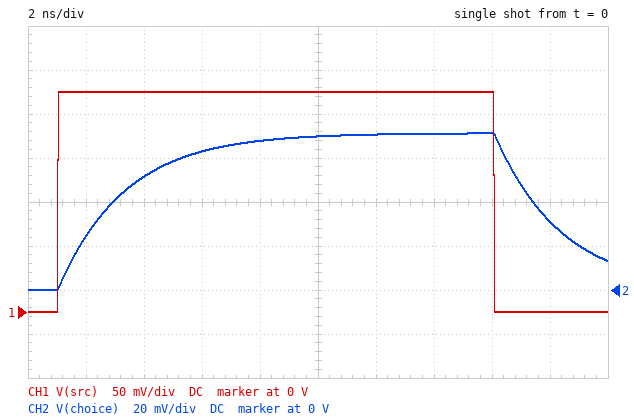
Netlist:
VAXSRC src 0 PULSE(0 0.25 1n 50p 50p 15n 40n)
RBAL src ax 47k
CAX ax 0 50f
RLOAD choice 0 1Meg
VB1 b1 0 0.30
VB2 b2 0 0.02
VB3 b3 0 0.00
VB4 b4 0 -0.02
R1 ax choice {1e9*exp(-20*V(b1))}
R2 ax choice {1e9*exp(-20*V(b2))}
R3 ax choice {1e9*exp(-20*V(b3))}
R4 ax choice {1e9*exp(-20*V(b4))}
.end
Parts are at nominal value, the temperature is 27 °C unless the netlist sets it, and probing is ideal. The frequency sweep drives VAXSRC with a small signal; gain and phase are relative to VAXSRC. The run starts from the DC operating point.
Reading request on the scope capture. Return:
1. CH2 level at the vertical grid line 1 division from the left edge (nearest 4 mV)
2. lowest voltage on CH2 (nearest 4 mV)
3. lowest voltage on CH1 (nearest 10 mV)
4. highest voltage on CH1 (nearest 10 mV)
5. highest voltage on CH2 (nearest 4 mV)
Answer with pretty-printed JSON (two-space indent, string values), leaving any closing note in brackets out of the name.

{
  "CH2 level at the vertical grid line 1 division from the left edge": "24 mV",
  "lowest voltage on CH2": "0 V",
  "lowest voltage on CH1": "0 V",
  "highest voltage on CH1": "250 mV",
  "highest voltage on CH2": "72 mV"
}
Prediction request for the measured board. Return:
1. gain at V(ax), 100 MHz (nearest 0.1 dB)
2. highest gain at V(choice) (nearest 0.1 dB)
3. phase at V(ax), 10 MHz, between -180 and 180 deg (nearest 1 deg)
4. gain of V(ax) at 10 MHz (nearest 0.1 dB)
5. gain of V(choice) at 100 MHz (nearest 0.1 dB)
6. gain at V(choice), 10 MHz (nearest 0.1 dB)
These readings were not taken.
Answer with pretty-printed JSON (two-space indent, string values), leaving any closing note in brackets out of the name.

{
  "gain at V(ax), 100 MHz": "-5.1 dB",
  "highest gain at V(choice)": "-10.9 dB",
  "phase at V(ax), 10 MHz, between -180 and 180 deg": "-8 deg",
  "gain of V(ax) at 10 MHz": "-0.2 dB",
  "gain of V(choice) at 100 MHz": "-15.8 dB",
  "gain at V(choice), 10 MHz": "-11.0 dB"
}
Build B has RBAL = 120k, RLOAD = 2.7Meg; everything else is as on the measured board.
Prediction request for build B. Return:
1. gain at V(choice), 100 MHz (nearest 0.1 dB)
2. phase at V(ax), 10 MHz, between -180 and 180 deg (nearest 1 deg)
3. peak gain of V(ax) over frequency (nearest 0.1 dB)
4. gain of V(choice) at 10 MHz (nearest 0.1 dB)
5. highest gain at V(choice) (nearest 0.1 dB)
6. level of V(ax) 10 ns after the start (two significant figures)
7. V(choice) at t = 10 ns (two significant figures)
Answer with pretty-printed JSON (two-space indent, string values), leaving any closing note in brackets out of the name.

{
  "gain at V(choice), 100 MHz": "-17.5 dB",
  "phase at V(ax), 10 MHz, between -180 and 180 deg": "-20 deg",
  "peak gain of V(ax) over frequency": "-0.2 dB",
  "gain of V(choice) at 10 MHz": "-6.4 dB",
  "highest gain at V(choice)": "-5.8 dB",
  "level of V(ax) 10 ns after the start": "190 mV",
  "V(choice) at t = 10 ns": "100 mV"
}
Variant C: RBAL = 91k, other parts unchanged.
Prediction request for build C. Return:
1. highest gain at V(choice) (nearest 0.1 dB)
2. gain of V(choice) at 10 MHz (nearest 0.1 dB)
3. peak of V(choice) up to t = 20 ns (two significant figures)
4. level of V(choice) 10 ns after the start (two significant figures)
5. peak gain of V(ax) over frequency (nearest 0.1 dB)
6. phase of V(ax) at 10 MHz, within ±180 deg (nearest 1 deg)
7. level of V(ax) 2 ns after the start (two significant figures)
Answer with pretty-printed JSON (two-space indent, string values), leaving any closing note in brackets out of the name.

{
  "highest gain at V(choice)": "-11.0 dB",
  "gain of V(choice) at 10 MHz": "-11.3 dB",
  "peak of V(choice) up to t = 20 ns": "68 mV",
  "level of V(choice) 10 ns after the start": "61 mV",
  "peak gain of V(ax) over frequency": "-0.2 dB",
  "phase of V(ax) at 10 MHz, within ±180 deg": "-16 deg",
  "level of V(ax) 2 ns after the start": "48 mV"
}
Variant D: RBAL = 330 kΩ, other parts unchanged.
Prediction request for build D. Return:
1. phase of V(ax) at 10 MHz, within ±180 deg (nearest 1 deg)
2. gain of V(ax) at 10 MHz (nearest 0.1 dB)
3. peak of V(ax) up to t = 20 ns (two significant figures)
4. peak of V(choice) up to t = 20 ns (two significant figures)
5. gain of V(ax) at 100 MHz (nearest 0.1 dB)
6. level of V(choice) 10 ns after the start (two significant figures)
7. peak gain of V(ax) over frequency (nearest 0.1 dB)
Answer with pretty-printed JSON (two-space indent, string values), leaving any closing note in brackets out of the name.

{
  "phase of V(ax) at 10 MHz, within ±180 deg": "-43 deg",
  "gain of V(ax) at 10 MHz": "-3.6 dB",
  "peak of V(ax) up to t = 20 ns": "140 mV",
  "peak of V(choice) up to t = 20 ns": "42 mV",
  "gain of V(ax) at 100 MHz": "-20.4 dB",
  "level of V(choice) 10 ns after the start": "30 mV",
  "peak gain of V(ax) over frequency": "-0.8 dB"
}
